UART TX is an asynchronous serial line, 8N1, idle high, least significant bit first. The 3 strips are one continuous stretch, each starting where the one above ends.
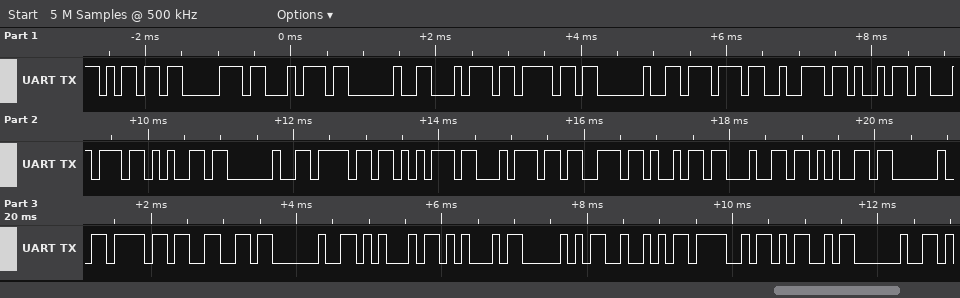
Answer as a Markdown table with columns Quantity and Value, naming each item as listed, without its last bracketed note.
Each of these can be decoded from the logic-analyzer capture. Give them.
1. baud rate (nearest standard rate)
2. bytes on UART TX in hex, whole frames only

| Quantity | Value |
|---|---|
| baud rate | 9600 baud |
| bytes on UART TX in hex, whole frames only | 6D 70 74 20 74 6F 20 77 72 69 74 65 20 6F 75 74 73 69 64 65 20 6F 66 20 45 45 50 52 4F 4D 20 |
